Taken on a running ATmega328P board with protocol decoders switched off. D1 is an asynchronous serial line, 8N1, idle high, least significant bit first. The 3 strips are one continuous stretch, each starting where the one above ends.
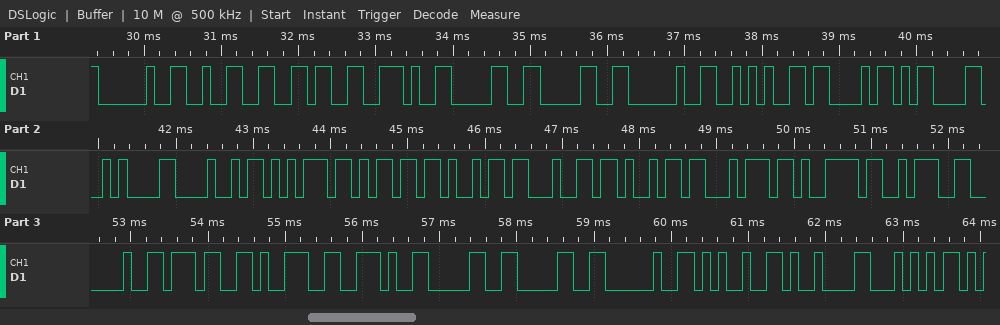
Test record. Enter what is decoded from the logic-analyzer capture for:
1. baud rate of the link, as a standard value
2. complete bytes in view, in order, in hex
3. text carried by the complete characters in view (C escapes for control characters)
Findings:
9600 baud
20 32 36 2E 30 30 20 2A 43 0D 0A 48 75 6D 69 64 69 74 79 3A 20 37 39 2E 30 30 20 25 09 54
" 26.00 *C\r\nHumidity: 79.00 %\tT"
